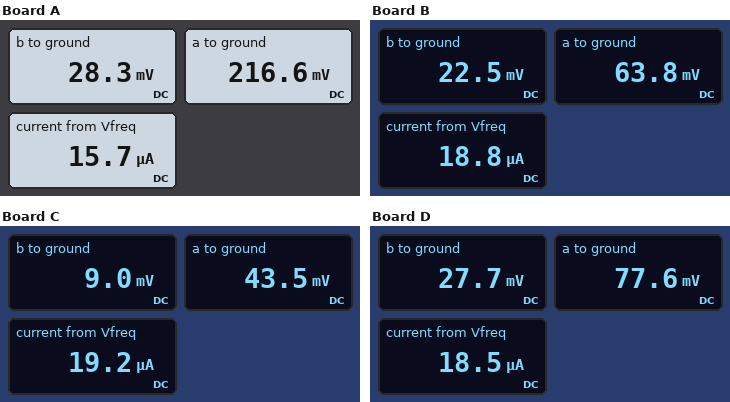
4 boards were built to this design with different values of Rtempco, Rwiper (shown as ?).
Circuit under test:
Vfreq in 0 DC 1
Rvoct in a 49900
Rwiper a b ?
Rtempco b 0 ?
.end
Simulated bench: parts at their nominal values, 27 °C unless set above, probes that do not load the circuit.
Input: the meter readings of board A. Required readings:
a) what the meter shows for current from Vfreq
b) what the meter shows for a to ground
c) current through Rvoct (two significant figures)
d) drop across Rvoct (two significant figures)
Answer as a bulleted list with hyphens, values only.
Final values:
- 15.7 µA
- 216.6 mV
- 16 µA
- 780 mV
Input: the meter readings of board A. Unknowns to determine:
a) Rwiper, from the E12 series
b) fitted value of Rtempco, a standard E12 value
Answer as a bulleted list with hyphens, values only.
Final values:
- 12 kΩ
- 1.8 kΩ
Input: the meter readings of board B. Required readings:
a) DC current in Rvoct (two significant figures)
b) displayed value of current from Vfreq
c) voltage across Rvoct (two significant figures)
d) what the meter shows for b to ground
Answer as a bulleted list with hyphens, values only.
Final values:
- 19 µA
- 18.8 µA
- 940 mV
- 22.5 mV
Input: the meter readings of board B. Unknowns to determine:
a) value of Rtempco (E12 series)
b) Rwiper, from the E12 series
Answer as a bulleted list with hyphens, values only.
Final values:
- 1.2 kΩ
- 2.2 kΩ
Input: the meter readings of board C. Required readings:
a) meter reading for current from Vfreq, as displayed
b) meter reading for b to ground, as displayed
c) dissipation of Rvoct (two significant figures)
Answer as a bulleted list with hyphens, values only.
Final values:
- 19.2 µA
- 9.0 mV
- 18 µW
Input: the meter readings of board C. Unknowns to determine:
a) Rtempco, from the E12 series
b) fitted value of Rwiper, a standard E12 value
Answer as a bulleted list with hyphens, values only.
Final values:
- 470 Ω
- 1.8 kΩ
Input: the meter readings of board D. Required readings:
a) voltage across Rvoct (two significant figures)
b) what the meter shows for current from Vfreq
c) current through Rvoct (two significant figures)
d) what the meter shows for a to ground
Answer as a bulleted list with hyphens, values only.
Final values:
- 920 mV
- 18.5 µA
- 18 µA
- 77.6 mV
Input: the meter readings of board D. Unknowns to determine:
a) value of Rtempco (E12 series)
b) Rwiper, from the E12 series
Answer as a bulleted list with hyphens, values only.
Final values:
- 1.5 kΩ
- 2.7 kΩ
